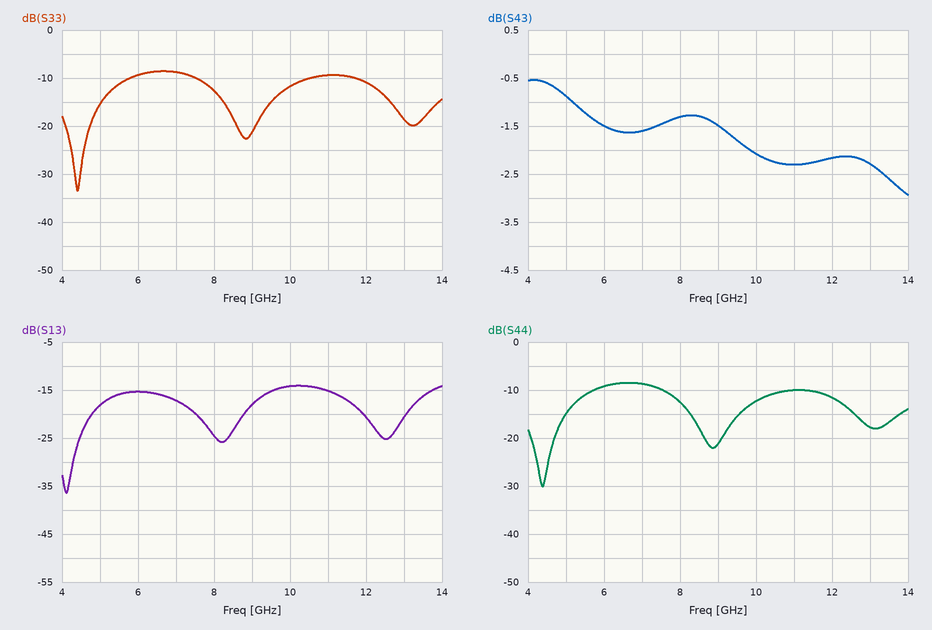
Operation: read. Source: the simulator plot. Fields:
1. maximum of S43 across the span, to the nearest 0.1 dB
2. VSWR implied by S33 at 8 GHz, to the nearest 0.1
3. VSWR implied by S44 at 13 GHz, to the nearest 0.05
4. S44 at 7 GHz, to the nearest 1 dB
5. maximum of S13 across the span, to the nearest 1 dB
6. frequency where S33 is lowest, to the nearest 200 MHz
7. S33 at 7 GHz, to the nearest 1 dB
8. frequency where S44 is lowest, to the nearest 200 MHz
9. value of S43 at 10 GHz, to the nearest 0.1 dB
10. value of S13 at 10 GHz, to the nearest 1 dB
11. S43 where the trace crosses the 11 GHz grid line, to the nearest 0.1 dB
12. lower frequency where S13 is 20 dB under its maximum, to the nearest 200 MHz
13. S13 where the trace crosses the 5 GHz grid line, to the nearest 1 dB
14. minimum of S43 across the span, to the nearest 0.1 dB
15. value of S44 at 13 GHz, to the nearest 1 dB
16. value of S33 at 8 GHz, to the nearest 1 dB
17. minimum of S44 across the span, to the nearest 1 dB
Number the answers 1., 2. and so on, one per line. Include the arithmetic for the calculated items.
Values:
1. -0.5 dB
2. |Γ| = 10^(-13/20) = 0.2239; VSWR = (1 + 0.2239)/(1 − 0.2239) ≈ 1.6
3. |Γ| = 10^(-18/20) = 0.1259; VSWR = (1 + 0.1259)/(1 − 0.1259) ≈ 1.29, so 1.30 to the nearest 0.05
4. -9 dB
5. -14 dB
6. 4.4 GHz
7. -9 dB
8. 4.4 GHz
9. -2.1 dB
10. -14 dB
11. -2.3 dB
12. 4.2 GHz
13. -18 dB
14. -2.9 dB
15. -18 dB
16. -13 dB
17. -30 dB
